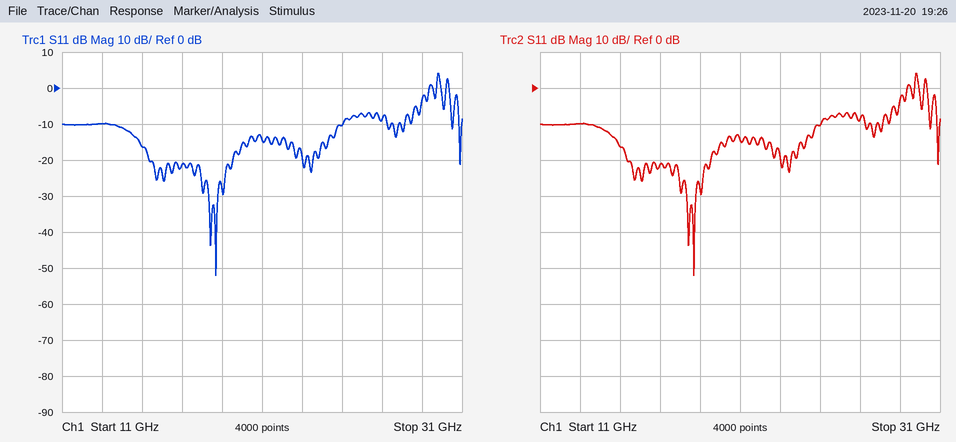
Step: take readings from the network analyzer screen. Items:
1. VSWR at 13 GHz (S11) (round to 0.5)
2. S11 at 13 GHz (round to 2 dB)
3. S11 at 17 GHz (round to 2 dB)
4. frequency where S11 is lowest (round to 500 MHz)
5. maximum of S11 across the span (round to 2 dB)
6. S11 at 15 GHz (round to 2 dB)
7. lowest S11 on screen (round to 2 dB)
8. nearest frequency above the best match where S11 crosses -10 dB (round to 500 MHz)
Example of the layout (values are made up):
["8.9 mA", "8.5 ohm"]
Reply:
["2.0", "-10 dB", "-22 dB", "18.5 GHz", "4 dB", "-16 dB", "-52 dB", "25.0 GHz"]
